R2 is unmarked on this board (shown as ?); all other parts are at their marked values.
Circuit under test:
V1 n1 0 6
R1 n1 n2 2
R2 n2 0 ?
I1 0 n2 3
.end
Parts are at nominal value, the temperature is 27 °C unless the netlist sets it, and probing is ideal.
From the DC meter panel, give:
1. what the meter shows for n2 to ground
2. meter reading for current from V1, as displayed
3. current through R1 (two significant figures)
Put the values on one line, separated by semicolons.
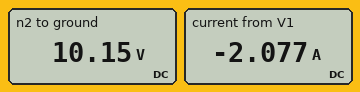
10.15 V; -2.077 A; 2.1 A
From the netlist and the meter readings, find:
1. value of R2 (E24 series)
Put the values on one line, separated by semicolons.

11 Ω
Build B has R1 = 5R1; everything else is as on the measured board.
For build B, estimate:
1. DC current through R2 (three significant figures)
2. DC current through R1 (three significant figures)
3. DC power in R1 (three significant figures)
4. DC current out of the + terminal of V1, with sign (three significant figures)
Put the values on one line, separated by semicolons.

1.32 A; 1.68 A; 14.3 W; -1.68 A
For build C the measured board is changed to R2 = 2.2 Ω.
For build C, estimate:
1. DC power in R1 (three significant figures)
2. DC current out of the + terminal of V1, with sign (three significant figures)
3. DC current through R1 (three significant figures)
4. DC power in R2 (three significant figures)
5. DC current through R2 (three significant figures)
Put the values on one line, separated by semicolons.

40.8 mW; -143 mA; 143 mA; 18.0 W; 2.86 A
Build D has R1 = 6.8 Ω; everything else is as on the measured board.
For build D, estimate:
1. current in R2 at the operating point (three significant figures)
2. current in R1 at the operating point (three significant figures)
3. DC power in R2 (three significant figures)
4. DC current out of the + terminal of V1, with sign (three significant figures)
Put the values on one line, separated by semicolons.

1.48 A; 1.52 A; 24.2 W; -1.52 A
